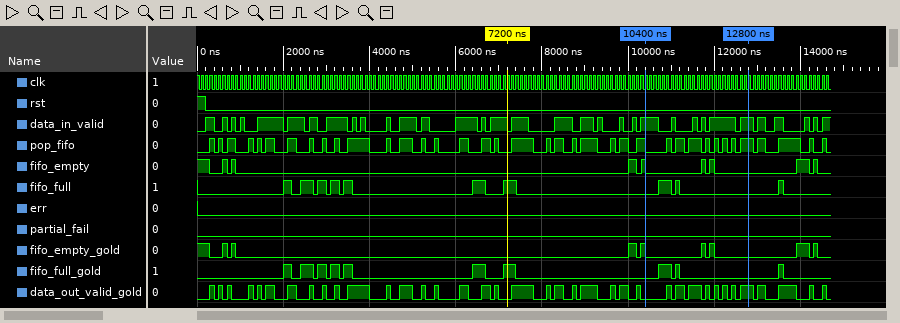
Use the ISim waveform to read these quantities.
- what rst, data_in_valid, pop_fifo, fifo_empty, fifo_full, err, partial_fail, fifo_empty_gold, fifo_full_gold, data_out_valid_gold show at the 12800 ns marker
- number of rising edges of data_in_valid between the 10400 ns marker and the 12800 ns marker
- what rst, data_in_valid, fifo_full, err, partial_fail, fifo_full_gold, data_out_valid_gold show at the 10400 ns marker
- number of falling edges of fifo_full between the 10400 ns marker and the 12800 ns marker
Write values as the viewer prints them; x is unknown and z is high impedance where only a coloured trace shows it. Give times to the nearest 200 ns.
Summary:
rst=0, data_in_valid=1, pop_fifo=1, fifo_empty=0, fifo_full=0, err=0, partial_fail=0, fifo_empty_gold=0, fifo_full_gold=0, data_out_valid_gold=1
5
rst=0, data_in_valid=1, fifo_full=0, err=0, partial_fail=0, fifo_full_gold=0, data_out_valid_gold=0
2
